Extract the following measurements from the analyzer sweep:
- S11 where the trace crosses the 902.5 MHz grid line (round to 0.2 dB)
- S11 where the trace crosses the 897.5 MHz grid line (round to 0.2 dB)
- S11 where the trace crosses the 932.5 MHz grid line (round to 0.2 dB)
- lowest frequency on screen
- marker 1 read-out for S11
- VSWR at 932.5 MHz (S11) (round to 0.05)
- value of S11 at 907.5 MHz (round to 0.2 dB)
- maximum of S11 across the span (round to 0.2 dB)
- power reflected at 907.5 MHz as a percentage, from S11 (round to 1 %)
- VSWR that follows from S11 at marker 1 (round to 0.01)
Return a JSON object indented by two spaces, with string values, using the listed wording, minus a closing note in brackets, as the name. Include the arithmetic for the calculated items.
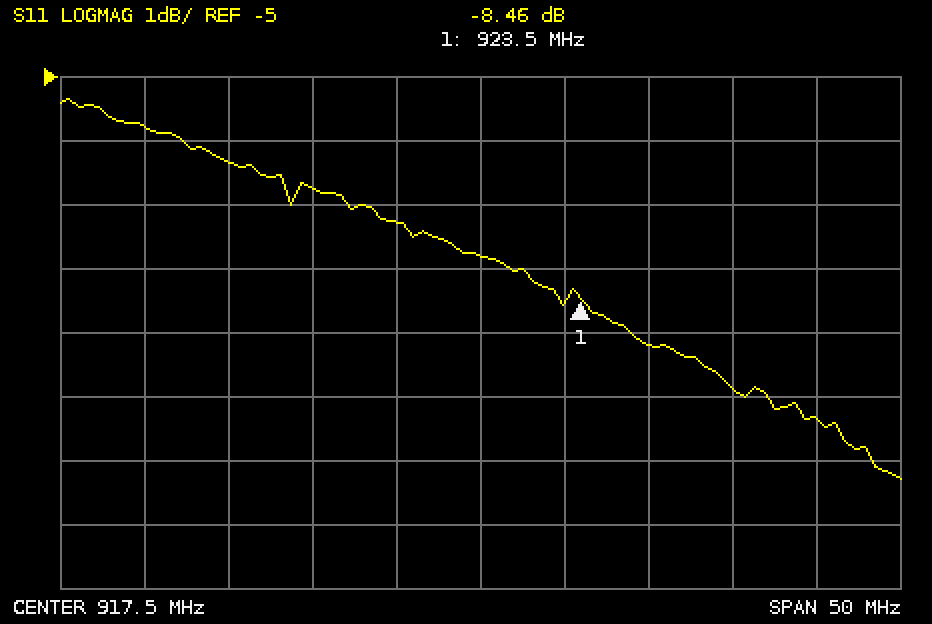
{
  "S11 where the trace crosses the 902.5 MHz grid line": "-6.4 dB",
  "S11 where the trace crosses the 897.5 MHz grid line": "-5.8 dB",
  "S11 where the trace crosses the 932.5 MHz grid line": "-9.8 dB",
  "lowest frequency on screen": "892.5 MHz",
  "marker 1 read-out for S11": "-8.46 dB",
  "VSWR at 932.5 MHz (S11)": "|Γ| = 10^(-9.8/20) = 0.3236; VSWR = (1 + 0.3236)/(1 − 0.3236) ≈ 1.96, so 1.95 to the nearest 0.05",
  "value of S11 at 907.5 MHz": "-6.8 dB",
  "maximum of S11 across the span": "-5.4 dB",
  "power reflected at 907.5 MHz as a percentage, from S11": "10^(-6.8/10) ≈ 21 %",
  "VSWR that follows from S11 at marker 1": "(1 + 0.3776)/(1 − 0.3776) ≈ 2.21"
}
